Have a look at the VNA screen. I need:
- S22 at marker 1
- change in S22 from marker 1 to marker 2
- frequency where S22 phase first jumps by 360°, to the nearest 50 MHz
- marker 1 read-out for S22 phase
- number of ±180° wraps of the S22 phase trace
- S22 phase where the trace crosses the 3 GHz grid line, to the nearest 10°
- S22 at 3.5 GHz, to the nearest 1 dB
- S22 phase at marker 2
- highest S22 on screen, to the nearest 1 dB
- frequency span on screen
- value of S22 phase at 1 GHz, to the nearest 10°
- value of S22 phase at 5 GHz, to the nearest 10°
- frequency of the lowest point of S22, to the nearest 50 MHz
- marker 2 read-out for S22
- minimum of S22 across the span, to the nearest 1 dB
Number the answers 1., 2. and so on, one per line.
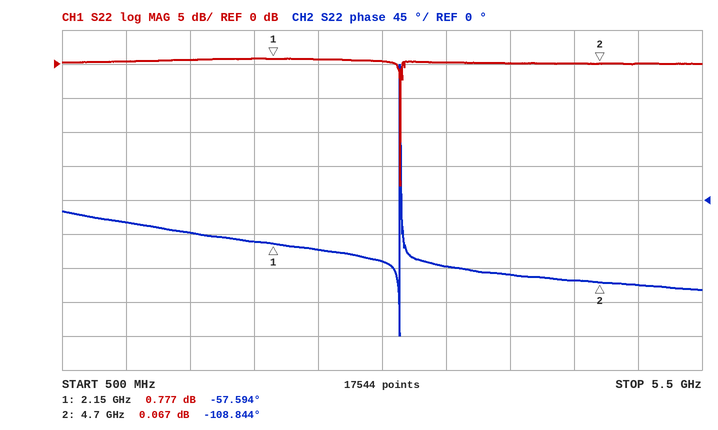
1. 0.777 dB
2. -0.710 dB
3. 3.15 GHz
4. -57.594°
5. 1
6. -80°
7. 0 dB
8. -108.844°
9. 1 dB
10. 5 GHz
11. -30°
12. -110°
13. 3.15 GHz
14. 0.067 dB
15. -18 dB
